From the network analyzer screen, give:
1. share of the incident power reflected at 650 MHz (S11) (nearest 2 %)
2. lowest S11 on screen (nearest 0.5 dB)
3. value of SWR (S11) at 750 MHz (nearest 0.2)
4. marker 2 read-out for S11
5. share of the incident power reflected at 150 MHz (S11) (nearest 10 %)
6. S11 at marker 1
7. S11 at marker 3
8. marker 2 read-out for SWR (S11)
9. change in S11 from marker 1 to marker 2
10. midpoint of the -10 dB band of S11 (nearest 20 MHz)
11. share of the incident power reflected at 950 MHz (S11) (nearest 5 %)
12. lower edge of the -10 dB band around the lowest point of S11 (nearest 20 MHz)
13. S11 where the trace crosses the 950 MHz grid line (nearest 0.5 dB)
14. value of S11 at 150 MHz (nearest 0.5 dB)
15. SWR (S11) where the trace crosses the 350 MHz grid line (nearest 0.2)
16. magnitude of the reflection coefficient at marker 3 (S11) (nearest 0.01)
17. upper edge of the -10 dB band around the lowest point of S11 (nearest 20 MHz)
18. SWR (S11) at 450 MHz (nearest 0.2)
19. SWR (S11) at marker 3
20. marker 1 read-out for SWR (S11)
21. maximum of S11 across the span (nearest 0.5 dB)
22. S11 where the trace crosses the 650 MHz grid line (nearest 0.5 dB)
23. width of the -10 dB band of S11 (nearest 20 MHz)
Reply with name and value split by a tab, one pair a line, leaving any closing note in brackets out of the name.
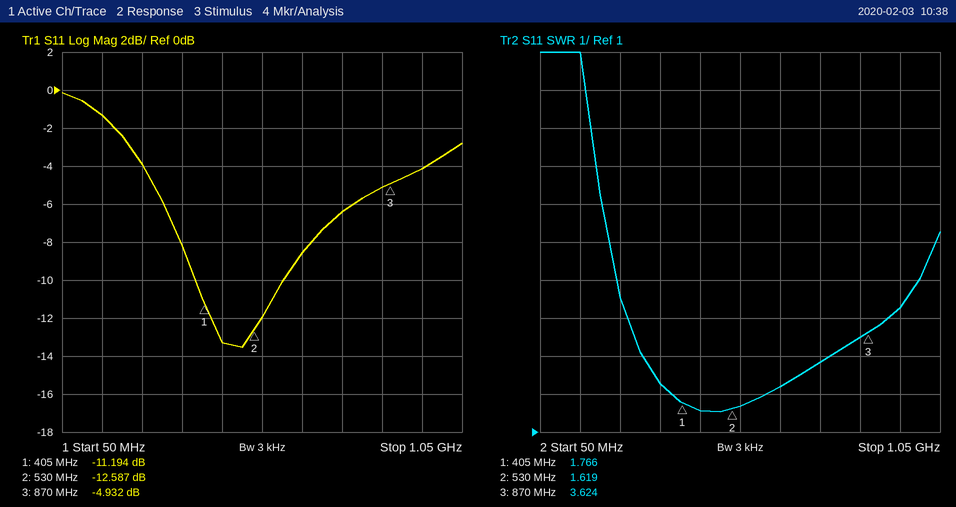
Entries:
share of the incident power reflected at 650 MHz (S11)	14 %
lowest S11 on screen	-13.5 dB
value of SWR (S11) at 750 MHz	2.8
marker 2 read-out for S11	-12.587 dB
share of the incident power reflected at 150 MHz (S11)	70 %
S11 at marker 1	-11.194 dB
S11 at marker 3	-4.932 dB
marker 2 read-out for SWR	1.619
change in S11 from marker 1 to marker 2	-1.393 dB
midpoint of the -10 dB band of S11	500 MHz
share of the incident power reflected at 950 MHz (S11)	40 %
lower edge of the -10 dB band around the lowest point of S11	380 MHz
S11 where the trace crosses the 950 MHz grid line	-4.0 dB
value of S11 at 150 MHz	-1.5 dB
SWR (S11) where the trace crosses the 350 MHz grid line	2.2
magnitude of the reflection coefficient at marker 3 (S11)	0.57
upper edge of the -10 dB band around the lowest point of S11	600 MHz
SWR (S11) at 450 MHz	1.6
SWR (S11) at marker 3	3.624
marker 1 read-out for SWR	1.766
maximum of S11 across the span	0.0 dB
S11 where the trace crosses the 650 MHz grid line	-8.5 dB
width of the -10 dB band of S11	220 MHz
